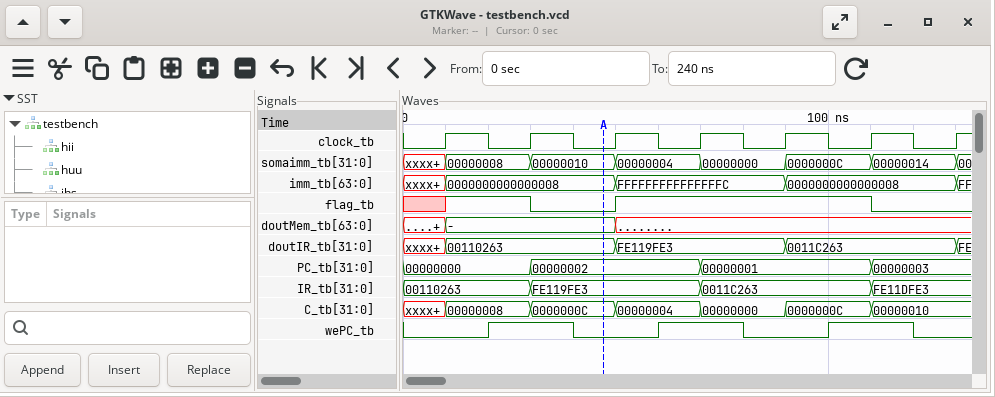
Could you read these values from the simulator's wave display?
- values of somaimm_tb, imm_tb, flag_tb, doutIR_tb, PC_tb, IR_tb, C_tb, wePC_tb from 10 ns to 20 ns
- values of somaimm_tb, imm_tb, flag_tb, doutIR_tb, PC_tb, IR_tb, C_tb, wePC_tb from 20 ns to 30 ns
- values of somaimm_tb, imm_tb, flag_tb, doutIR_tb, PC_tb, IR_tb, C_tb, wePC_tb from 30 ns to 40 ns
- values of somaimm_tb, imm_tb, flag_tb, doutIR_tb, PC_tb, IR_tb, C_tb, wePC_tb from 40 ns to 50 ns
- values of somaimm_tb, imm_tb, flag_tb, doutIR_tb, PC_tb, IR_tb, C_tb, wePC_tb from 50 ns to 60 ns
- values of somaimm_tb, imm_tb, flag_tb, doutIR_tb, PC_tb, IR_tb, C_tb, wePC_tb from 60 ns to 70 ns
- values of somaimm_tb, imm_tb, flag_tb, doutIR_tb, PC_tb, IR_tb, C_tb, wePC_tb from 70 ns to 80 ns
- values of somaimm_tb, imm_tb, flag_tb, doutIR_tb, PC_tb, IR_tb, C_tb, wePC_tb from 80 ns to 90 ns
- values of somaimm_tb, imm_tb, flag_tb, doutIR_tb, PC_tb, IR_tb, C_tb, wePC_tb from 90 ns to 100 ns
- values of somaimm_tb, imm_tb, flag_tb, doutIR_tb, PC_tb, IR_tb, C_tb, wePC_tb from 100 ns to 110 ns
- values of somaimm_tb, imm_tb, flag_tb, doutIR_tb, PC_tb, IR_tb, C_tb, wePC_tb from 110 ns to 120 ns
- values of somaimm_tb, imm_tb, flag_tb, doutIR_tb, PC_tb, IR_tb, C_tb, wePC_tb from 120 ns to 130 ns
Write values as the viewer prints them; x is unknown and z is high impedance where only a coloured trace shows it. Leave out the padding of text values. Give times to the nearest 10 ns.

somaimm_tb=00000008, imm_tb=0000000000000008, flag_tb=1, doutIR_tb=00110263, PC_tb=00000000, IR_tb=00110263, C_tb=00000008, wePC_tb=0
somaimm_tb=00000008, imm_tb=0000000000000008, flag_tb=1, doutIR_tb=00110263, PC_tb=00000000, IR_tb=00110263, C_tb=00000008, wePC_tb=1
somaimm_tb=00000010, imm_tb=0000000000000008, flag_tb=0, doutIR_tb=00110263, PC_tb=00000002, IR_tb=FE119FE3, C_tb=0000000C, wePC_tb=1
somaimm_tb=00000010, imm_tb=0000000000000008, flag_tb=0, doutIR_tb=00110263, PC_tb=00000002, IR_tb=FE119FE3, C_tb=0000000C, wePC_tb=0
somaimm_tb=00000004, imm_tb=FFFFFFFFFFFFFFFC, flag_tb=1, doutIR_tb=FE119FE3, PC_tb=00000002, IR_tb=FE119FE3, C_tb=00000004, wePC_tb=0
somaimm_tb=00000004, imm_tb=FFFFFFFFFFFFFFFC, flag_tb=1, doutIR_tb=FE119FE3, PC_tb=00000002, IR_tb=FE119FE3, C_tb=00000004, wePC_tb=1
somaimm_tb=00000000, imm_tb=FFFFFFFFFFFFFFFC, flag_tb=1, doutIR_tb=FE119FE3, PC_tb=00000001, IR_tb=0011C263, C_tb=00000000, wePC_tb=1
somaimm_tb=00000000, imm_tb=FFFFFFFFFFFFFFFC, flag_tb=1, doutIR_tb=FE119FE3, PC_tb=00000001, IR_tb=0011C263, C_tb=00000000, wePC_tb=0
somaimm_tb=0000000C, imm_tb=0000000000000008, flag_tb=1, doutIR_tb=0011C263, PC_tb=00000001, IR_tb=0011C263, C_tb=0000000C, wePC_tb=0
somaimm_tb=0000000C, imm_tb=0000000000000008, flag_tb=1, doutIR_tb=0011C263, PC_tb=00000001, IR_tb=0011C263, C_tb=0000000C, wePC_tb=1
somaimm_tb=00000014, imm_tb=0000000000000008, flag_tb=0, doutIR_tb=0011C263, PC_tb=00000003, IR_tb=FE11DFE3, C_tb=00000010, wePC_tb=1
somaimm_tb=00000014, imm_tb=0000000000000008, flag_tb=0, doutIR_tb=0011C263, PC_tb=00000003, IR_tb=FE11DFE3, C_tb=00000010, wePC_tb=0
